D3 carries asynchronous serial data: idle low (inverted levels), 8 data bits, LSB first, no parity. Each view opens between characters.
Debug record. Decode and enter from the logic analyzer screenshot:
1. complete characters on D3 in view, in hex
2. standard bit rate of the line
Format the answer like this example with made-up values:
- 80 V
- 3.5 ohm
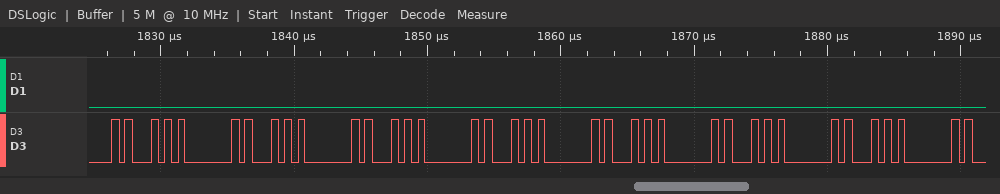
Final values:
- 5D, 7F, 57, 5D, 7F, 57, 5D, 7F, 57, 5D, 7F
- 2000000 baud
